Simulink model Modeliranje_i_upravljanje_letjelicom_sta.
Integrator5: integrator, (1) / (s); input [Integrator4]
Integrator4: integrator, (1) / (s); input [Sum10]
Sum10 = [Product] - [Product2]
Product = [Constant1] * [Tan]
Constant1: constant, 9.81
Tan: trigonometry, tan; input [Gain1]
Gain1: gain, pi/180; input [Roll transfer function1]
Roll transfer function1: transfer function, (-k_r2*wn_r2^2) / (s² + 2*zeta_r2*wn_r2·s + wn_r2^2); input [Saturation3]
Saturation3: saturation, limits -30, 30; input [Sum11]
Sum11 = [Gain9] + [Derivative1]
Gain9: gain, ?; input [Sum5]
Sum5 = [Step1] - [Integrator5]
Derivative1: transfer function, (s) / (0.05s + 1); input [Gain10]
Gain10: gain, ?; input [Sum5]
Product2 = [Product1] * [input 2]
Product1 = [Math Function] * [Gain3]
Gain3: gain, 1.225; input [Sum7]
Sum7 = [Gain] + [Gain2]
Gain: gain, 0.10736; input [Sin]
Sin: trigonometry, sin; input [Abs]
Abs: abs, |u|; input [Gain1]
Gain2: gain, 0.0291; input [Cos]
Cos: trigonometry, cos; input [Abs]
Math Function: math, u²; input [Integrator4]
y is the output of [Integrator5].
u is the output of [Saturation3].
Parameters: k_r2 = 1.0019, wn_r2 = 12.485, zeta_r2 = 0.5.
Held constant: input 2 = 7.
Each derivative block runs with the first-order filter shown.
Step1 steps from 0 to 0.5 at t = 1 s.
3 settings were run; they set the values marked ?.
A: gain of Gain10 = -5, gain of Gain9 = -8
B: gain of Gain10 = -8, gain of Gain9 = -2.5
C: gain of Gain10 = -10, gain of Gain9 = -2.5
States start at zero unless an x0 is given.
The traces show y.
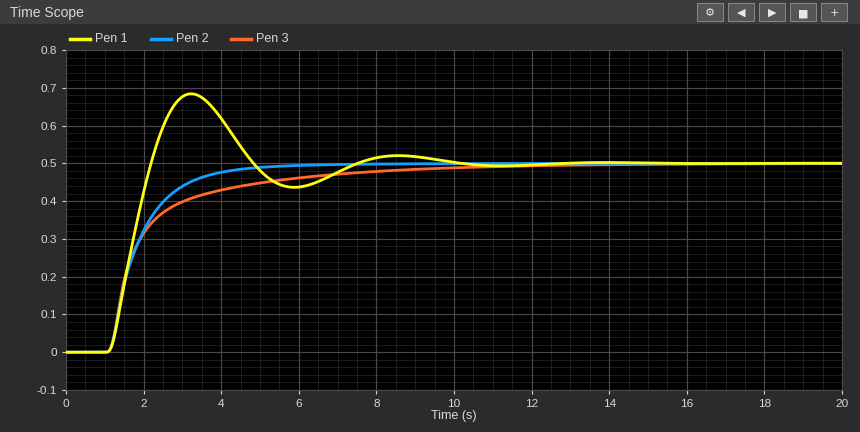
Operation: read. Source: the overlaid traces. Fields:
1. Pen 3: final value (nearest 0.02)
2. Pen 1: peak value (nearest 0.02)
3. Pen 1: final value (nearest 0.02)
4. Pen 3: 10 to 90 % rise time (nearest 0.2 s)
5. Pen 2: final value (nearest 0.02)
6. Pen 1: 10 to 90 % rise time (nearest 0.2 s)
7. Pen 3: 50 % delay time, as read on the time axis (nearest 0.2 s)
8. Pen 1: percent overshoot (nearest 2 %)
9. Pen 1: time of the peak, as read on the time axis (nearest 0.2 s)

0.50
0.68
0.50
3.8 s
0.50
0.8 s
1.6 s
36 %
3.2 s
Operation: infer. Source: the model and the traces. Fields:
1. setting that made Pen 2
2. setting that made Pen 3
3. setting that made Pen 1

B
C
A
